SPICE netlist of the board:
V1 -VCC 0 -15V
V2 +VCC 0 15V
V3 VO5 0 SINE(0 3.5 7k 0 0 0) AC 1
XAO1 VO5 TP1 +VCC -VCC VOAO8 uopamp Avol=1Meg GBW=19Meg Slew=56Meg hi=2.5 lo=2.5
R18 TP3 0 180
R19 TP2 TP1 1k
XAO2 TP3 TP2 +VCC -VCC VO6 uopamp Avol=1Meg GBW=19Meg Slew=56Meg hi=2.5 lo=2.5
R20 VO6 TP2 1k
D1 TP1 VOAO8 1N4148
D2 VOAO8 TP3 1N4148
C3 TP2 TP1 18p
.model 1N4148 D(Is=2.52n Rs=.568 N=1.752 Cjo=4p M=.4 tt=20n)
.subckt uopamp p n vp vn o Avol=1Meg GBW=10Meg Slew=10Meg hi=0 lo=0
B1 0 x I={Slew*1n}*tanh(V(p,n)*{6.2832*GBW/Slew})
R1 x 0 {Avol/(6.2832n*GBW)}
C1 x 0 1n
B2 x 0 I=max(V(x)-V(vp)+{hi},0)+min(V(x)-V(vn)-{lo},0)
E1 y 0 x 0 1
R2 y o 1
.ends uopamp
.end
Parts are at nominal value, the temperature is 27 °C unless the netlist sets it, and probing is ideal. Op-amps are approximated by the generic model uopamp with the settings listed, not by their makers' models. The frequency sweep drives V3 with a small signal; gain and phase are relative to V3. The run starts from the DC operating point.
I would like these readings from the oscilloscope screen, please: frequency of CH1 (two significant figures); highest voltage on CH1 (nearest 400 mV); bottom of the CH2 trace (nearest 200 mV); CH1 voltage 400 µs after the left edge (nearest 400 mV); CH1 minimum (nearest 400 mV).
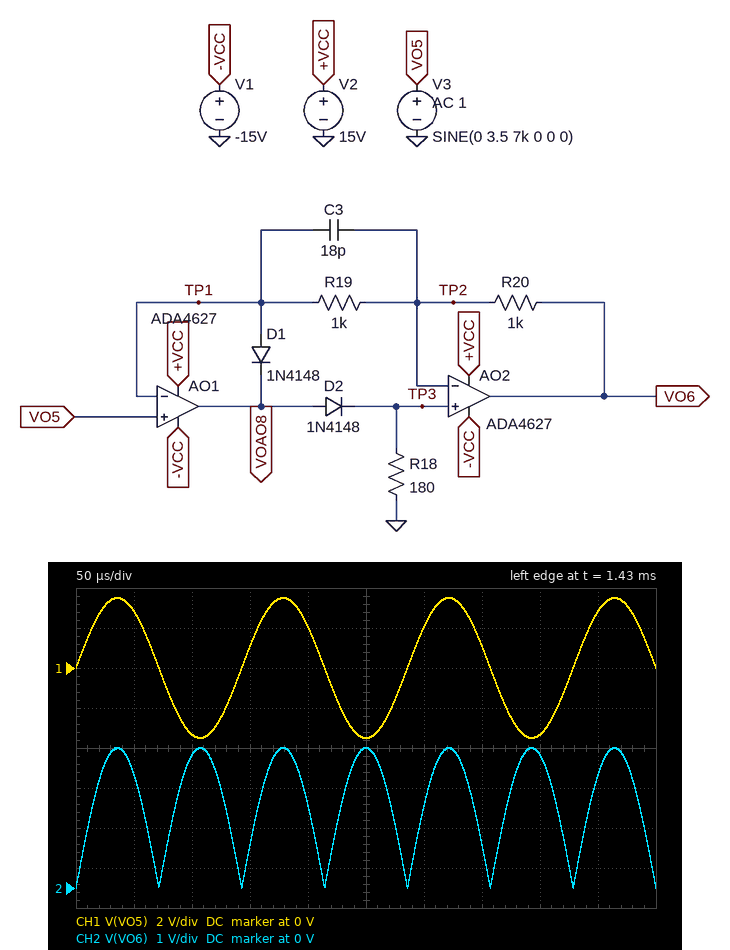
7.0 kHz
3.6 V
0 V
-3.2 V
-3.6 V
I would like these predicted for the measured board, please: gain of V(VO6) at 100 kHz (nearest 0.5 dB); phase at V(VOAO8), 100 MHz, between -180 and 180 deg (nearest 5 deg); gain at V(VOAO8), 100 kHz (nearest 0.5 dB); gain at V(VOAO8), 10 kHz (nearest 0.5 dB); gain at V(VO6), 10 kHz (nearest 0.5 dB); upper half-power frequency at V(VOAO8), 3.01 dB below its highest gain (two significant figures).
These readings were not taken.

-12.0 dB
-80 deg
41.5 dB
61.5 dB
-12.0 dB
810 Hz
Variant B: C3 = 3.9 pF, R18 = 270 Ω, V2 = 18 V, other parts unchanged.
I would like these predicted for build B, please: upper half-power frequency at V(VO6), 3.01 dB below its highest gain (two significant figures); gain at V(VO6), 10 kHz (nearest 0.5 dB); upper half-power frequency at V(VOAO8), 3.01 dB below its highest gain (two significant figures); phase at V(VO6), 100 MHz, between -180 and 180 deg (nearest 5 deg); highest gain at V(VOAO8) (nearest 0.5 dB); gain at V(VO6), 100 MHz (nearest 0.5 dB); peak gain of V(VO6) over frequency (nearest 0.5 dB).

1.0 kHz
-13.0 dB
850 Hz
0 deg
83.0 dB
-39.0 dB
-5.0 dB
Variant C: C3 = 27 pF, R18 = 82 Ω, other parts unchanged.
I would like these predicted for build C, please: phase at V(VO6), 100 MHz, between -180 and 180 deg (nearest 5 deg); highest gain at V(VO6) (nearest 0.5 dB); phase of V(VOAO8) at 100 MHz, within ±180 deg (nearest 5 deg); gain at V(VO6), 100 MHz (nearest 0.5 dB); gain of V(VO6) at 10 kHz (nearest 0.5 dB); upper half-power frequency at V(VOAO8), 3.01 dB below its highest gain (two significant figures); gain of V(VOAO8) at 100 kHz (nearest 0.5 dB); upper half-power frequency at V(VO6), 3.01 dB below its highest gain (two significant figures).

25 deg
-1.5 dB
-80 deg
-31.0 dB
-10.5 dB
770 Hz
42.0 dB
880 Hz
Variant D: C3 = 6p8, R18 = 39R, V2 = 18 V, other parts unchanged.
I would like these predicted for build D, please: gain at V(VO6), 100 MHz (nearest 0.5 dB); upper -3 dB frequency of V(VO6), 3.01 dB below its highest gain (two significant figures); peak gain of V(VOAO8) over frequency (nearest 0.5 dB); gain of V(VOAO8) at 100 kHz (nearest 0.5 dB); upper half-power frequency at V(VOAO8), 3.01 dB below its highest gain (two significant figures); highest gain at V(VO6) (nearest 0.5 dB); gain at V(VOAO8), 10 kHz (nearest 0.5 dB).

-31.0 dB
850 Hz
84.5 dB
42.0 dB
750 Hz
-1.0 dB
62.0 dB
